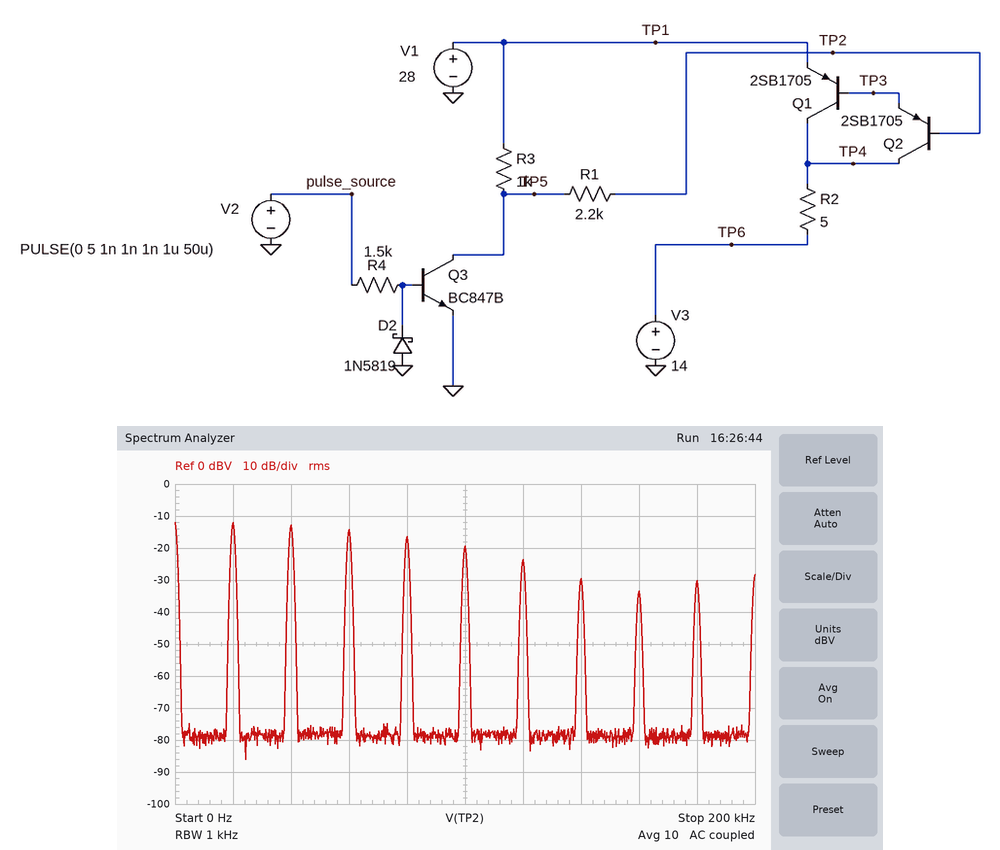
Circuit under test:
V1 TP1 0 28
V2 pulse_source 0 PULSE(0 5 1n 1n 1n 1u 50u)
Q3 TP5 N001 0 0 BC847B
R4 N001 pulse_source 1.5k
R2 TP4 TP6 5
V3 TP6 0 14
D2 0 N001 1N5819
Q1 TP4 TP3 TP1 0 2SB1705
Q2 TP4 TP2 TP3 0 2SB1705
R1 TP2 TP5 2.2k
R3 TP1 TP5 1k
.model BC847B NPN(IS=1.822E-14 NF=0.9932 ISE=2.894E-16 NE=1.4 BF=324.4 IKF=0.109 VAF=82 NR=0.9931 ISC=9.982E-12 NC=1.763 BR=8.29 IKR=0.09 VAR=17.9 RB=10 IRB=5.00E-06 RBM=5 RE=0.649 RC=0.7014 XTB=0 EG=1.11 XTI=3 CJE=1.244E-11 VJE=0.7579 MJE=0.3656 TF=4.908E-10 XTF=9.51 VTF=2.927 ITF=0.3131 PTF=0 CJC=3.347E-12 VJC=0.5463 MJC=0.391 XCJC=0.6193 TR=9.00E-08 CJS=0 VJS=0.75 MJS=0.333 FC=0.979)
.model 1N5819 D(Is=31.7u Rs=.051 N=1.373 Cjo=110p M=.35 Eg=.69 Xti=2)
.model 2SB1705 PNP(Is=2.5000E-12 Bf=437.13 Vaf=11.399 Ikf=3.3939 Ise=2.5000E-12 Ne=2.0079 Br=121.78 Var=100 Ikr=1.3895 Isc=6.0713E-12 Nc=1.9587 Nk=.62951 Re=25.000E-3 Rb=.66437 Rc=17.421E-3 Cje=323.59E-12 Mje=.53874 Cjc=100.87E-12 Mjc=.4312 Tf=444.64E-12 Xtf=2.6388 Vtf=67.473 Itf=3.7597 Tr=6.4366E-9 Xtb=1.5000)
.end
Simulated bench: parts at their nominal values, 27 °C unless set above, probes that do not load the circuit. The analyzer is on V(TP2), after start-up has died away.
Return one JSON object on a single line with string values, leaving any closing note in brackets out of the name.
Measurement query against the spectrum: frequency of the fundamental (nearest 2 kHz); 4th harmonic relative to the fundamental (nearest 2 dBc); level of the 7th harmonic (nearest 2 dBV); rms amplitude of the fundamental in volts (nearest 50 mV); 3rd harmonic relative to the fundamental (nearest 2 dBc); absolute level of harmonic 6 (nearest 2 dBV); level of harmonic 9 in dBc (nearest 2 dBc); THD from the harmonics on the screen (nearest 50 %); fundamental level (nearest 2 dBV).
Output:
{"frequency of the fundamental": "20 kHz", "4th harmonic relative to the fundamental": "-4 dBc", "level of the 7th harmonic": "-30 dBV", "rms amplitude of the fundamental in volts": "250 mV", "3rd harmonic relative to the fundamental": "-2 dBc", "absolute level of harmonic 6": "-24 dBV", "level of harmonic 9 in dBc": "-18 dBc", "THD from the harmonics on the screen": "150 %", "fundamental level": "-12 dBV"}
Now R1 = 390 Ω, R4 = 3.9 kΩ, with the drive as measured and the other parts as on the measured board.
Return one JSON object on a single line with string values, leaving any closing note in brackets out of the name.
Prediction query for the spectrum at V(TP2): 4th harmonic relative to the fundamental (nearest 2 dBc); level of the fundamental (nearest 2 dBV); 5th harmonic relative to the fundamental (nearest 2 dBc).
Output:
{"4th harmonic relative to the fundamental": "-2 dBc", "level of the fundamental": "-14 dBV", "5th harmonic relative to the fundamental": "-4 dBc"}
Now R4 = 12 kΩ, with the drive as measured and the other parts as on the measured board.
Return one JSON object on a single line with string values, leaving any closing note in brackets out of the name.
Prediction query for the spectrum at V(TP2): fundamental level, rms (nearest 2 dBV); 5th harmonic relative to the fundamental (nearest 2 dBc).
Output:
{"fundamental level, rms": "-14 dBV", "5th harmonic relative to the fundamental": "-6 dBc"}
